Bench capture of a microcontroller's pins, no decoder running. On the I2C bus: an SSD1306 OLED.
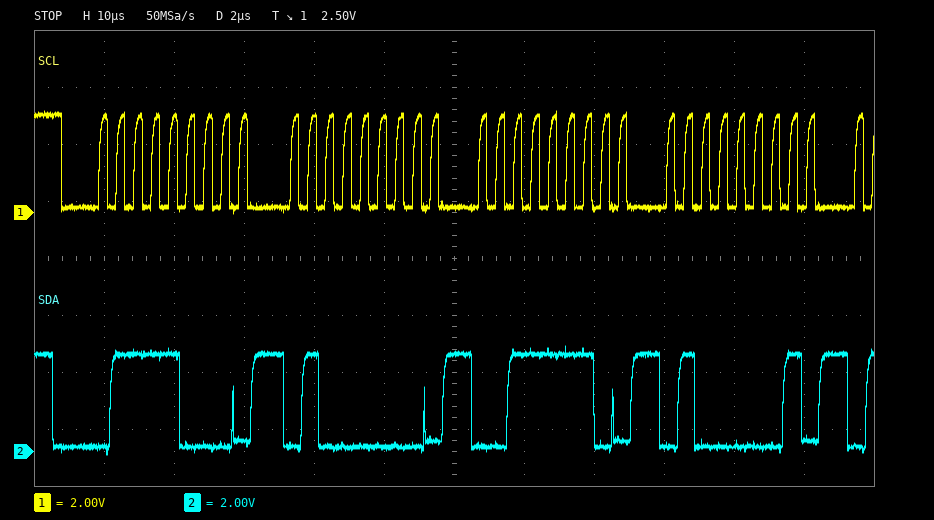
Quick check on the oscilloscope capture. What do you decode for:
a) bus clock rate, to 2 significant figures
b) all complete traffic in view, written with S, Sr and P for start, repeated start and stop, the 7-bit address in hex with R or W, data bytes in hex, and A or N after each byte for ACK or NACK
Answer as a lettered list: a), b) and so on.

a) 400 kHz
b) S 3CW A 40 A 3E A 41 A
